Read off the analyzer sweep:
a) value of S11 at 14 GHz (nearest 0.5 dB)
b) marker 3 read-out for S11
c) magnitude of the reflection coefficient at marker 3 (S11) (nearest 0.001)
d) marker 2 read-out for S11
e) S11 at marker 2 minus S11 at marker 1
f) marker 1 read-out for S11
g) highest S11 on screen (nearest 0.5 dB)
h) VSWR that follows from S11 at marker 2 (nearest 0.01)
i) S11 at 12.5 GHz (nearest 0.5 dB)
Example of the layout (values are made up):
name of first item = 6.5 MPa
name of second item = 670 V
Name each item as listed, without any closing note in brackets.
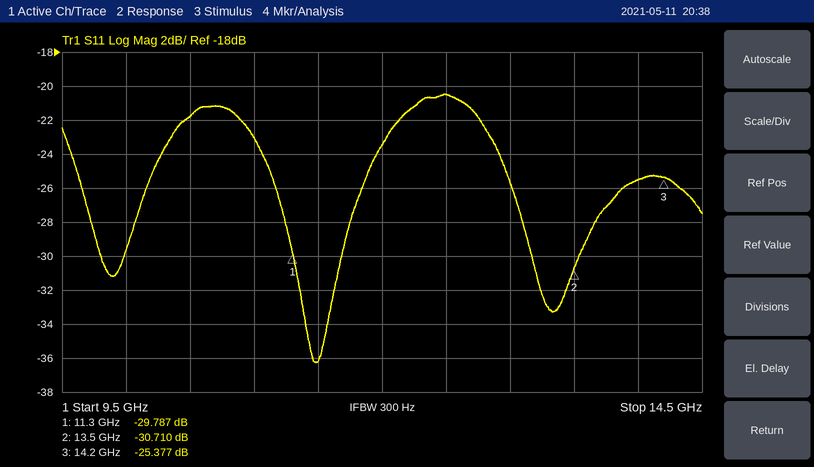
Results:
value of S11 at 14 GHz = -25.5 dB
marker 3 read-out for S11 = -25.377 dB
magnitude of the reflection coefficient at marker 3 (S11) = 0.054
marker 2 read-out for S11 = -30.710 dB
S11 at marker 2 minus S11 at marker 1 = -0.923 dB
marker 1 read-out for S11 = -29.787 dB
highest S11 on screen = -20.5 dB
VSWR that follows from S11 at marker 2 = 1.06
S11 at 12.5 GHz = -20.5 dB
